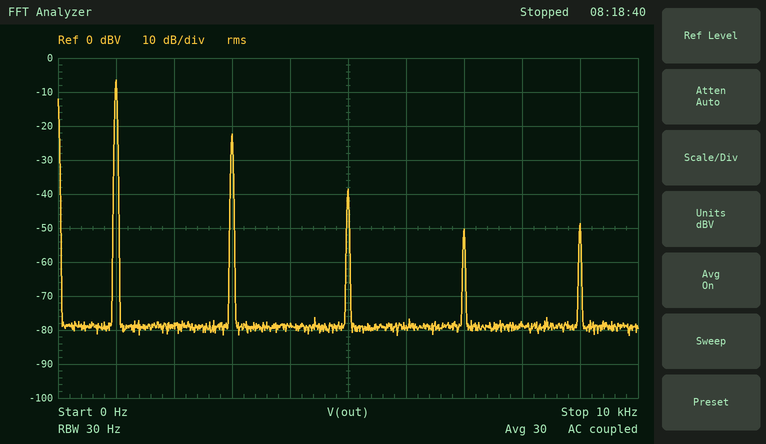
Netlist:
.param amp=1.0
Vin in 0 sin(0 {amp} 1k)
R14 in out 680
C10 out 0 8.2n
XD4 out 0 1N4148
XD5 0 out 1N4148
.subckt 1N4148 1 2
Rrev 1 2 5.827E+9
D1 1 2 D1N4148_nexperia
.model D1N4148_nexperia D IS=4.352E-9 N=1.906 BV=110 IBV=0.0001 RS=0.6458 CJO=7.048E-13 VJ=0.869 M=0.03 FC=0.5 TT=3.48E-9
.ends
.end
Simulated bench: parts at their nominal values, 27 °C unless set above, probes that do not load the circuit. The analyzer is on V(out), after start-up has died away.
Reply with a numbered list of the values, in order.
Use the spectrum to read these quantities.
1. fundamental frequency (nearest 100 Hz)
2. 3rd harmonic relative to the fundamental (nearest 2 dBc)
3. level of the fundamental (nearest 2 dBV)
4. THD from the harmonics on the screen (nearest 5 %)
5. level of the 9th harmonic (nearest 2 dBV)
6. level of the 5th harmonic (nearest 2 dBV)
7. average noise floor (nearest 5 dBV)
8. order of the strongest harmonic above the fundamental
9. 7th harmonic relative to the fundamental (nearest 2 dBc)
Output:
1. 1.0 kHz
2. -16 dBc
3. -6 dBV
4. 15 %
5. -48 dBV
6. -38 dBV
7. -80 dBV
8. 3
9. -44 dBc
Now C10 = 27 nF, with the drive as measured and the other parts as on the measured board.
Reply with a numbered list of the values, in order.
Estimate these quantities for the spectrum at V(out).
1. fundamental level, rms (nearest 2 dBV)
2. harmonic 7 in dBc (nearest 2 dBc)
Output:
1. -6 dBV
2. -42 dBc
